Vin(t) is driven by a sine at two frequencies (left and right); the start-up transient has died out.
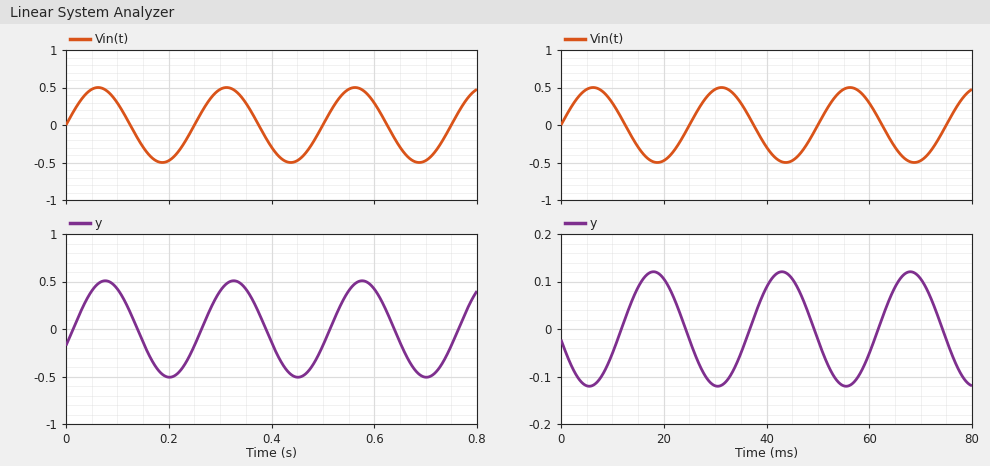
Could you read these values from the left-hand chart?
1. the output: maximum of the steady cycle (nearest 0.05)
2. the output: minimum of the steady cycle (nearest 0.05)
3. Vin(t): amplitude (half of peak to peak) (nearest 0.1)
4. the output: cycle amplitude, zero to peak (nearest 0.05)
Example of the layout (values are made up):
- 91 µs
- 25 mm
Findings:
- 0.50
- -0.50
- 0.5
- 0.50
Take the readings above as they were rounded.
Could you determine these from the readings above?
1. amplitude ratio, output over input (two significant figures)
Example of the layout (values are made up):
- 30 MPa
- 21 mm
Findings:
- 1.0
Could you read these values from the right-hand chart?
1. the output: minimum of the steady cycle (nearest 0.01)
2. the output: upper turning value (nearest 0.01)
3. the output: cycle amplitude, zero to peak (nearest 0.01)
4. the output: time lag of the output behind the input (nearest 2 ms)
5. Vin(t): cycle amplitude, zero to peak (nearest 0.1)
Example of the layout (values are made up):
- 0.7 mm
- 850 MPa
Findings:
- -0.12
- 0.12
- 0.12
- 12 ms
- 0.5
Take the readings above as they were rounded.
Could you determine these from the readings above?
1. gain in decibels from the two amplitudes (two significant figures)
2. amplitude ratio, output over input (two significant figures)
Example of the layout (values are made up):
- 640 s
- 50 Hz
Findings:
- -12 dB
- 0.24
